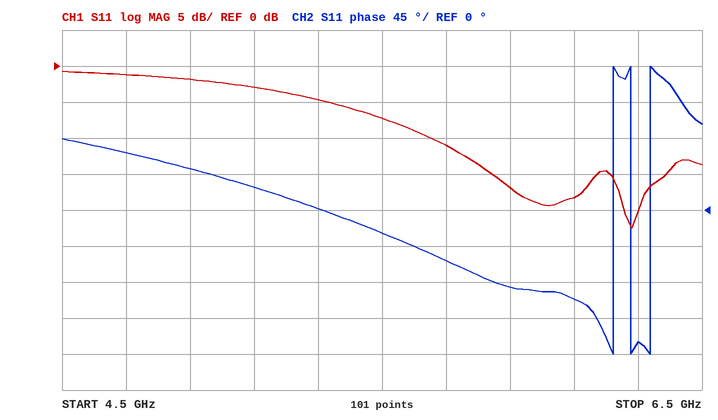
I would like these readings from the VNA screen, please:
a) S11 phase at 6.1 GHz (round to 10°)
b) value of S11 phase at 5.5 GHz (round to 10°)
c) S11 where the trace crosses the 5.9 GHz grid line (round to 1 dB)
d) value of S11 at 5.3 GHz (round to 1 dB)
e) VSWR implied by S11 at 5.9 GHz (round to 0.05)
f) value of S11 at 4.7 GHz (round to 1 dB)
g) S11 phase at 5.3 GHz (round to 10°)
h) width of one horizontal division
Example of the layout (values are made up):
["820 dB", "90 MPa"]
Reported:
["-110°", "-30°", "-17 dB", "-5 dB", "1.35", "-1 dB", "0°", "200 MHz"]
